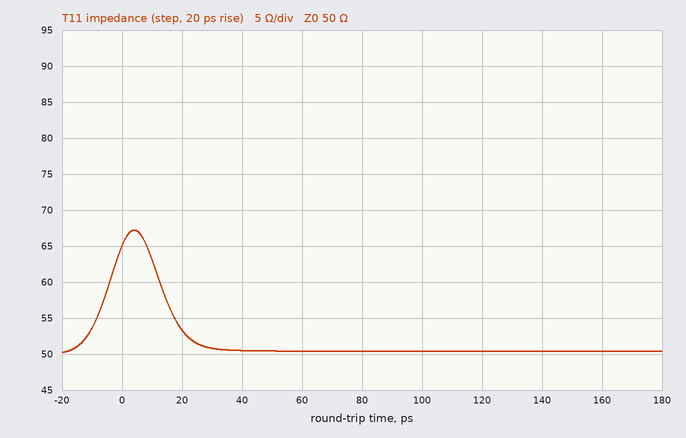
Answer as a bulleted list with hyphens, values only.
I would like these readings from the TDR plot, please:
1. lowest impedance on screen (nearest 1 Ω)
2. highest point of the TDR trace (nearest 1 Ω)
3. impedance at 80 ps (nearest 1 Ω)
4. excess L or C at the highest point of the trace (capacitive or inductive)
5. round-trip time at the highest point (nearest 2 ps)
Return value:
- 50 Ω
- 67 Ω
- 50 Ω
- inductive
- 4 ps
